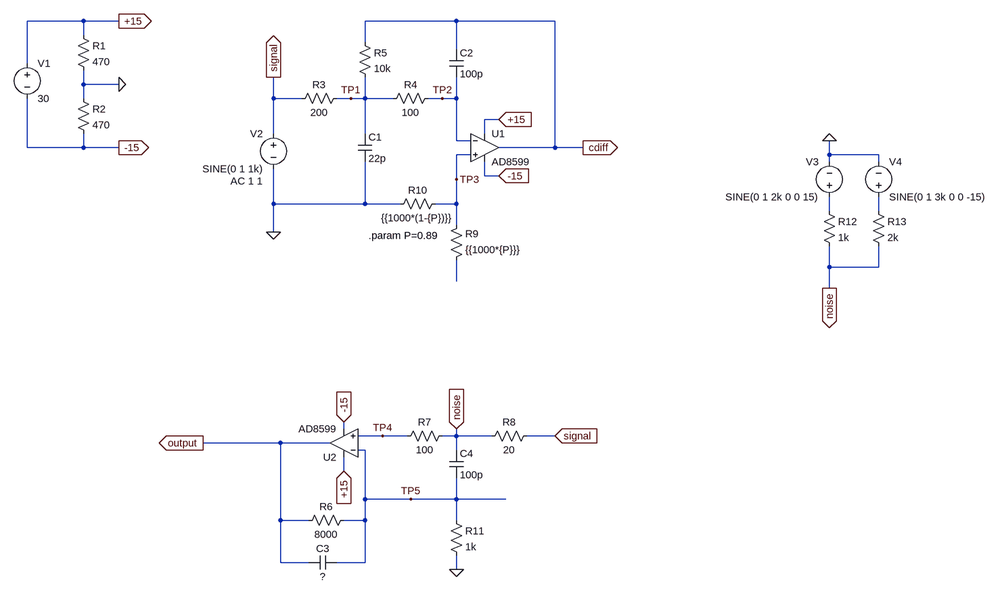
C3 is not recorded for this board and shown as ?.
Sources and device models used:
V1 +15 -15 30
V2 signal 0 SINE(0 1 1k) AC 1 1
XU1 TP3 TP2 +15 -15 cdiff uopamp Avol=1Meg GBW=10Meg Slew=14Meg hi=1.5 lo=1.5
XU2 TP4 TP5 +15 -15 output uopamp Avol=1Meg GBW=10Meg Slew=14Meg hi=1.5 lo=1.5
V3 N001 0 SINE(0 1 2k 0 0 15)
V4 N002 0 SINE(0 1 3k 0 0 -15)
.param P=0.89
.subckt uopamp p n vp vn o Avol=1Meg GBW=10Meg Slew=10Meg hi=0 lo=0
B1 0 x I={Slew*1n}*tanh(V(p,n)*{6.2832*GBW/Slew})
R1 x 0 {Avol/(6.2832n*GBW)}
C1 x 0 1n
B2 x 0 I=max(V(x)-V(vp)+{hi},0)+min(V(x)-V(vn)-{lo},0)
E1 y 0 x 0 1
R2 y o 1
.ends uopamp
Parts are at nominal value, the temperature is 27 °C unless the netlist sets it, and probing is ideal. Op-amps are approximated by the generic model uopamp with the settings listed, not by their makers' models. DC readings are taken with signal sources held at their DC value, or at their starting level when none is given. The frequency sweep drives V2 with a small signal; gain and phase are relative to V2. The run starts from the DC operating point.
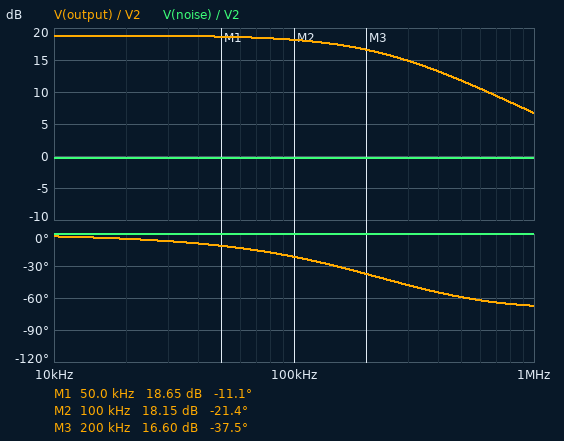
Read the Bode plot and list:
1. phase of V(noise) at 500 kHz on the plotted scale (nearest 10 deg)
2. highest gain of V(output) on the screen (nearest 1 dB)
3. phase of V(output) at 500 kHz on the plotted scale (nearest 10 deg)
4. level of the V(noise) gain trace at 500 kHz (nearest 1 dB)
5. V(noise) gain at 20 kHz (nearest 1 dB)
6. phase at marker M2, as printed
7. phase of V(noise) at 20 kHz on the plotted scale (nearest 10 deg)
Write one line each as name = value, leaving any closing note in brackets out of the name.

phase of V(noise) at 500 kHz on the plotted scale = 0 deg
highest gain of V(output) on the screen = 19 dB
phase of V(output) at 500 kHz on the plotted scale = -60 deg
level of the V(noise) gain trace at 500 kHz = 0 dB
V(noise) gain at 20 kHz = 0 dB
phase at marker M2, as printed = -21.4 deg
phase of V(noise) at 20 kHz on the plotted scale = 0 deg
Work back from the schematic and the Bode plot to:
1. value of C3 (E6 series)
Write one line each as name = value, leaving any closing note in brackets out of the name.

value of C3 = 68 pF
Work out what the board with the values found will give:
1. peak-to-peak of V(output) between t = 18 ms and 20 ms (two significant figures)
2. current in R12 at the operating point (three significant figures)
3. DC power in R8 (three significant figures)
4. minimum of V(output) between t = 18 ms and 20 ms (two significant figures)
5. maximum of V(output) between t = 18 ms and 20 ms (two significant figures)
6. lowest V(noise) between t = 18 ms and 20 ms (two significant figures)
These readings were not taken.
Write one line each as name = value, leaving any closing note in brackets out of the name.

peak-to-peak of V(output) between t = 18 ms and 20 ms = 17 V
current in R12 at the operating point = 256 µA
DC power in R8 = 316 nW
minimum of V(output) between t = 18 ms and 20 ms = -8.7 V
maximum of V(output) between t = 18 ms and 20 ms = 8.6 V
lowest V(noise) between t = 18 ms and 20 ms = -970 mV
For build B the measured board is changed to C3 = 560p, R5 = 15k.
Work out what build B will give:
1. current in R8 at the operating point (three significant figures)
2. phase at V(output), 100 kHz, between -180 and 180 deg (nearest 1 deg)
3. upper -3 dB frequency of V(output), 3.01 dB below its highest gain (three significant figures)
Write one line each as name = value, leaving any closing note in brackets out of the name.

current in R8 at the operating point = 126 µA
phase at V(output), 100 kHz, between -180 and 180 deg = -54 deg
upper -3 dB frequency of V(output), 3.01 dB below its highest gain = 35.0 kHz
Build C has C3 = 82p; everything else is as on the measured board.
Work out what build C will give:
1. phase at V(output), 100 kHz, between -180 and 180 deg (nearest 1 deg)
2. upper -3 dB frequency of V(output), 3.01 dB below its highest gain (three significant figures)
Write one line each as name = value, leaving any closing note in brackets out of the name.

phase at V(output), 100 kHz, between -180 and 180 deg = -24 deg
upper -3 dB frequency of V(output), 3.01 dB below its highest gain = 209 kHz
